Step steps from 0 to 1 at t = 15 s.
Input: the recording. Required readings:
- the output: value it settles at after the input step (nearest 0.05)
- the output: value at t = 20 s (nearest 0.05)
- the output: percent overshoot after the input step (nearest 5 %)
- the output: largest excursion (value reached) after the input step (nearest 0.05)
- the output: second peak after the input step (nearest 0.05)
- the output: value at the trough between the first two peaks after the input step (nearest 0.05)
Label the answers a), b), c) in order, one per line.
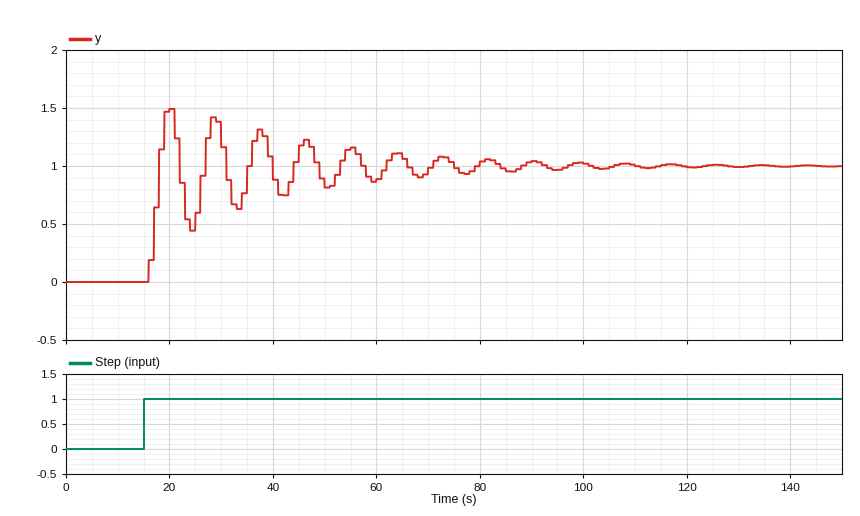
a) 1.00
b) 1.50
c) 50 %
d) 1.50
e) 1.40
f) 0.45
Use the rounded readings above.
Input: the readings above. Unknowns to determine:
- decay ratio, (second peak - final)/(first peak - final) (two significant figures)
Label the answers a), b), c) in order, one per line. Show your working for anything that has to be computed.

a) (1.4 - 1) / (1.5 - 1) = 0.80
